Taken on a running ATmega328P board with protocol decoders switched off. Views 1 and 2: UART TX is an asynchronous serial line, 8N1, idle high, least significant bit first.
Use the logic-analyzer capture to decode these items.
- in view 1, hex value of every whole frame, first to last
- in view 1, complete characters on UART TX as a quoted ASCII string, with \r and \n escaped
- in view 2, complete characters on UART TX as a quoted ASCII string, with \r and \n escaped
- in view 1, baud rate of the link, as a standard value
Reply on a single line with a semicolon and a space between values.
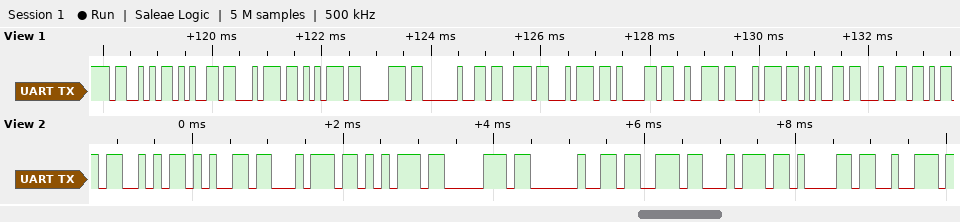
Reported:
0x53 0x65 0x74 0x75 0x70 0x20 0x73 0x74 0x61 0x72 0x74 0x65 0x64; "Setup started"; "Setup star"; 9600 baud
